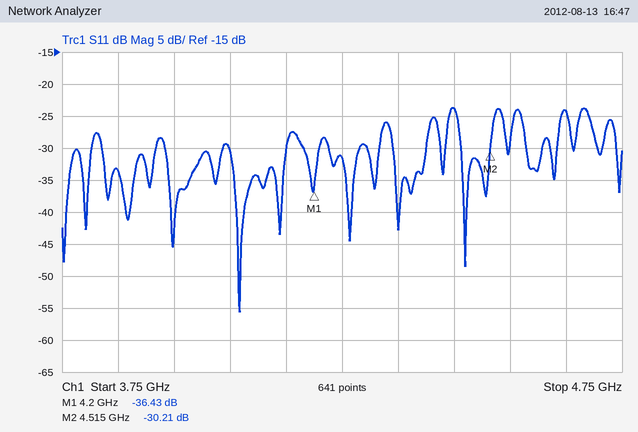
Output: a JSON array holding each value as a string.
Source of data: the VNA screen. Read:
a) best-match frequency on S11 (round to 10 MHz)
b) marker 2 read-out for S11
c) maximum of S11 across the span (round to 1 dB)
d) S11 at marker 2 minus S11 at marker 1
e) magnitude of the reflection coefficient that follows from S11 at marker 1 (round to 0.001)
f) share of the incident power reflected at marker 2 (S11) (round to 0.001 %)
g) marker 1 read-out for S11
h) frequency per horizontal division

["4.07 GHz", "-30.21 dB", "-24 dB", "6.22 dB", "0.015", "0.095 %", "-36.43 dB", "100 MHz"]
